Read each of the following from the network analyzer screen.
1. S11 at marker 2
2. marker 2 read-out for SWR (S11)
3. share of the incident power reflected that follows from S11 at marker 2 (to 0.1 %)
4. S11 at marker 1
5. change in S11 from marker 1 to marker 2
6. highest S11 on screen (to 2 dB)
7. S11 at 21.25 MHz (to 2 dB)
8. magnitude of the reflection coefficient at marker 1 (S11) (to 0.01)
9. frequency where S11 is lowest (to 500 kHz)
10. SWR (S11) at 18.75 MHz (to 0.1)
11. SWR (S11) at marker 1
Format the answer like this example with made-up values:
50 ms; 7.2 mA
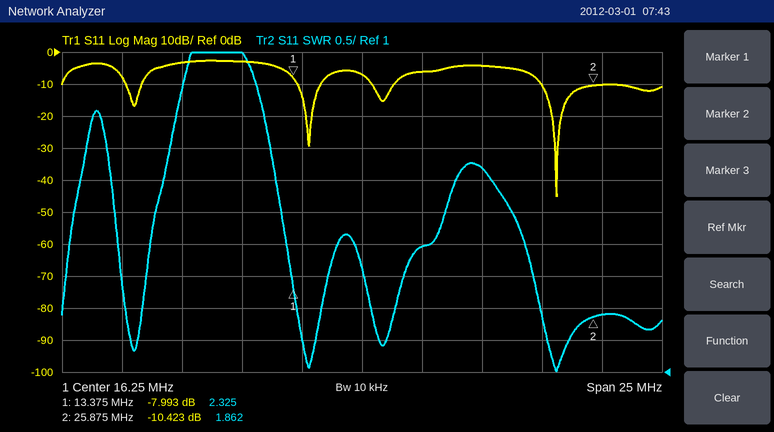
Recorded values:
-10.423 dB; 1.862; 9.1 %; -7.993 dB; -2.430 dB; -2 dB; -4 dB; 0.40; 24.5 MHz; 3.0; 2.325
